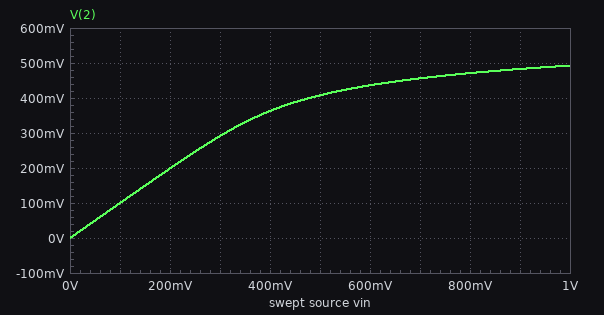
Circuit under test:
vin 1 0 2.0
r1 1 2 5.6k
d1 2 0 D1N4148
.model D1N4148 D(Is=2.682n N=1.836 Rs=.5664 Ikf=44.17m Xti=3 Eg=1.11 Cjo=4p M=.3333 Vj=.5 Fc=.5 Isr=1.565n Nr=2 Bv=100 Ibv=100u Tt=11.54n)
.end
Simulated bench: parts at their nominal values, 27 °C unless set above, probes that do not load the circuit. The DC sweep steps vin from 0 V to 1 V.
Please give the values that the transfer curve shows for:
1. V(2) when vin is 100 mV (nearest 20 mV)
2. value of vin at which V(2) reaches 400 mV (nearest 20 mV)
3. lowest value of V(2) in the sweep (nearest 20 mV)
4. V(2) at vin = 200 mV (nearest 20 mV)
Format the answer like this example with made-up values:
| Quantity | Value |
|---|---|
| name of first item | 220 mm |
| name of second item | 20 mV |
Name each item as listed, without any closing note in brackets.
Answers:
| Quantity | Value |
|---|---|
| V(2) when vin is 100 mV | 100 mV |
| value of vin at which V(2) reaches 400 mV | 480 mV |
| lowest value of V(2) in the sweep | 0 V |
| V(2) at vin = 200 mV | 200 mV |
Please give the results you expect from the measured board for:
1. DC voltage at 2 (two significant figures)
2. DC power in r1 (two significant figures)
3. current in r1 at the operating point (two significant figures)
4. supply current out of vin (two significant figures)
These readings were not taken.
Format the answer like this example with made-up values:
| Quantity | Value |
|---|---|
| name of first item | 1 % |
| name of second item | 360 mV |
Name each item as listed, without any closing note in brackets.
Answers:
| Quantity | Value |
|---|---|
| DC voltage at 2 | 540 mV |
| DC power in r1 | 380 µW |
| current in r1 at the operating point | 260 µA |
| supply current out of vin | 260 µA |
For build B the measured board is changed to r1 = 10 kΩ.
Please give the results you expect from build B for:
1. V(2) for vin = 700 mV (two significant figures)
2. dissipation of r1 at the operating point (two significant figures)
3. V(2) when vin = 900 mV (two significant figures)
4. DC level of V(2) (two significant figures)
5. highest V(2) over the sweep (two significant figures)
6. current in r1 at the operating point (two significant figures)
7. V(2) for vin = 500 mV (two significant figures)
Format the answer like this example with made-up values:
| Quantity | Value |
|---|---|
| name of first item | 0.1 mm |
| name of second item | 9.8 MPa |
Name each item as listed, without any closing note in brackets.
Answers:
| Quantity | Value |
|---|---|
| V(2) for vin = 700 mV | 430 mV |
| dissipation of r1 at the operating point | 220 µW |
| V(2) when vin = 900 mV | 460 mV |
| DC level of V(2) | 520 mV |
| highest V(2) over the sweep | 470 mV |
| current in r1 at the operating point | 150 µA |
| V(2) for vin = 500 mV | 390 mV |
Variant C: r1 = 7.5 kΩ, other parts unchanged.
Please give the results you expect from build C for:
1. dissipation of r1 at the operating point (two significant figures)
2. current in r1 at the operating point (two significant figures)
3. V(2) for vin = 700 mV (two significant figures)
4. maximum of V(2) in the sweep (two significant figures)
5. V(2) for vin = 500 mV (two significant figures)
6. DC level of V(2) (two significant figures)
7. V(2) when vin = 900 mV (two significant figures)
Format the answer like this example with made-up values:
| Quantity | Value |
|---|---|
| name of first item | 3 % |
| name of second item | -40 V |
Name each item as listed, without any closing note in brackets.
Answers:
| Quantity | Value |
|---|---|
| dissipation of r1 at the operating point | 290 µW |
| current in r1 at the operating point | 200 µA |
| V(2) for vin = 700 mV | 440 mV |
| maximum of V(2) in the sweep | 480 mV |
| V(2) for vin = 500 mV | 400 mV |
| DC level of V(2) | 530 mV |
| V(2) when vin = 900 mV | 470 mV |
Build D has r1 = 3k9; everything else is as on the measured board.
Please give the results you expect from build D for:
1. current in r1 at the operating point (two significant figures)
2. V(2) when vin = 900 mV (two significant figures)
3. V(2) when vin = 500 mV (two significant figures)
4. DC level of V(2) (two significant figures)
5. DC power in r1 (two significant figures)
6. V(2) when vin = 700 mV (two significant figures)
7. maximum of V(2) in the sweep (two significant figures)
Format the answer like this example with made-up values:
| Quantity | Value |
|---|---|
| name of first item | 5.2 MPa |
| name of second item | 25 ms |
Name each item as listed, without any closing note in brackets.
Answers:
| Quantity | Value |
|---|---|
| current in r1 at the operating point | 370 µA |
| V(2) when vin = 900 mV | 500 mV |
| V(2) when vin = 500 mV | 420 mV |
| DC level of V(2) | 560 mV |
| DC power in r1 | 530 µW |
| V(2) when vin = 700 mV | 470 mV |
| maximum of V(2) in the sweep | 510 mV |
